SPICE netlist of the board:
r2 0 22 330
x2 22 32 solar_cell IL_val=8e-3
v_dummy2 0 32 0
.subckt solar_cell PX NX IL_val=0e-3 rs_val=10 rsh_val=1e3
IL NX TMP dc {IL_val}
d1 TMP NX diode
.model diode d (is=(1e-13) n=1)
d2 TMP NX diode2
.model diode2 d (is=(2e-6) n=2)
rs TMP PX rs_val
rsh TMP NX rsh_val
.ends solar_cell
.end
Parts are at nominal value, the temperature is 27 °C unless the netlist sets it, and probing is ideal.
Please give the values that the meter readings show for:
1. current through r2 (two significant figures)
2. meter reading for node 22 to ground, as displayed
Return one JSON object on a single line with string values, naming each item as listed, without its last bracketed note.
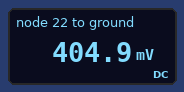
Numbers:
{"current through r2": "1.2 mA", "meter reading for node 22 to ground, as displayed": "404.9 mV"}
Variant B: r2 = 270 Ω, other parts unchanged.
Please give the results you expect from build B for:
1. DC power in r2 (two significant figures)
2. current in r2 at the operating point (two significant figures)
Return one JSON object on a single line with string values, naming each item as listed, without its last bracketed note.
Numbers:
{"DC power in r2": "590 µW", "current in r2 at the operating point": "1.5 mA"}
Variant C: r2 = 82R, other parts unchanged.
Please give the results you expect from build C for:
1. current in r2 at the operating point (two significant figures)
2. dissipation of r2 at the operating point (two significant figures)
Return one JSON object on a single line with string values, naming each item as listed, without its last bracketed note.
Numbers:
{"current in r2 at the operating point": "4.2 mA", "dissipation of r2 at the operating point": "1.4 mW"}
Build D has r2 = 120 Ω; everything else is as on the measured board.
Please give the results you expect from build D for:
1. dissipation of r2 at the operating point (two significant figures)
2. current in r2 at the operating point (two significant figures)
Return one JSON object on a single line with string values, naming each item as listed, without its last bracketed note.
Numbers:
{"dissipation of r2 at the operating point": "1.1 mW", "current in r2 at the operating point": "3.1 mA"}
